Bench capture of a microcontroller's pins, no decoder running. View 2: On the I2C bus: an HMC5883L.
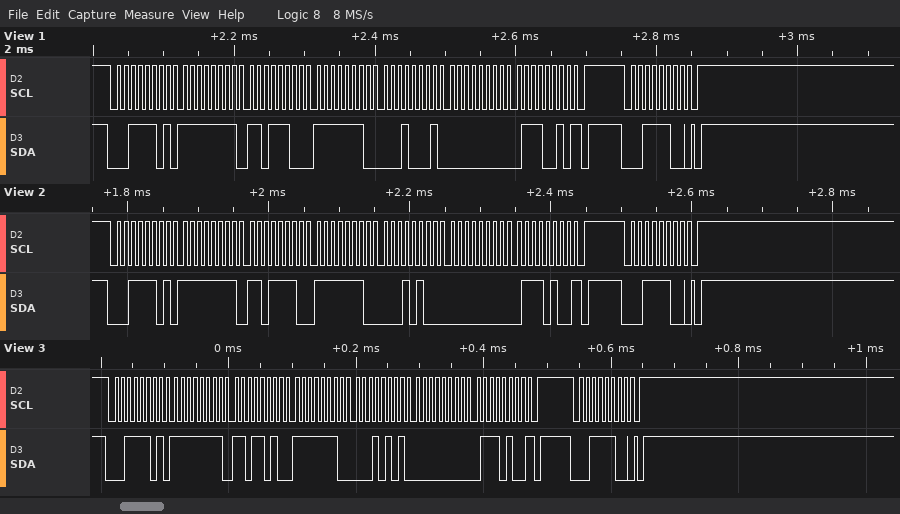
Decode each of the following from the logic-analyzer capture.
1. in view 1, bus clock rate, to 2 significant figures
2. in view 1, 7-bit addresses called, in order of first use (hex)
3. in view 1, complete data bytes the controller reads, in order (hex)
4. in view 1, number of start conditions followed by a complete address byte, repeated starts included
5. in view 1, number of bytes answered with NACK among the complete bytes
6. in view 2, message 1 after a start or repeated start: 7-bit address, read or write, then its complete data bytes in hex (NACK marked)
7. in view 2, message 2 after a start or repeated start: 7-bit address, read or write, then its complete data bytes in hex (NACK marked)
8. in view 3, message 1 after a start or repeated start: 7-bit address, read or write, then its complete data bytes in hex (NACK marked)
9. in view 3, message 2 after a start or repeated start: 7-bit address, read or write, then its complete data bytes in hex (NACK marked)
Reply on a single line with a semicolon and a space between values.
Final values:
100 kHz; 0x1E; FF DC FE 11 00 72; 2; 1; 0x1E read: FF DE FE 14 00 74 NACK; 0x1E write; 0x1E read: FF DA FE 15 00 74 NACK; 0x1E write
